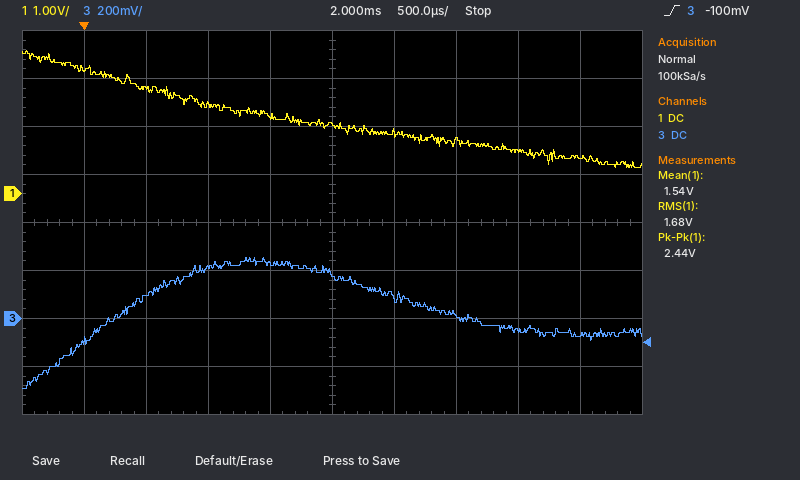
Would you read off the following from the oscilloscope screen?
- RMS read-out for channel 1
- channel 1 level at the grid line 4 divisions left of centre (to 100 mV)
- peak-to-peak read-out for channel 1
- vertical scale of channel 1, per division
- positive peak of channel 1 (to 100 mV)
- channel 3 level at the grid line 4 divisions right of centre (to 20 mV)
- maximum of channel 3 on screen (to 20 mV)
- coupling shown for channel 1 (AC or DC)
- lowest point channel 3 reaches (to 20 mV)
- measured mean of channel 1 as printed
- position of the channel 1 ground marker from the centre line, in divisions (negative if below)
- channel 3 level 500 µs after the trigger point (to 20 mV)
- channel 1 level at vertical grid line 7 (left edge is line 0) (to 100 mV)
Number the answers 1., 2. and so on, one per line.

1. 1.68 V
2. 2.6 V
3. 2.44 V
4. 1 V
5. 3.0 V
6. -60 mV
7. 260 mV
8. DC
9. -300 mV
10. 1.54 V
11. +0.6 div
12. 100 mV
13. 1.1 V
